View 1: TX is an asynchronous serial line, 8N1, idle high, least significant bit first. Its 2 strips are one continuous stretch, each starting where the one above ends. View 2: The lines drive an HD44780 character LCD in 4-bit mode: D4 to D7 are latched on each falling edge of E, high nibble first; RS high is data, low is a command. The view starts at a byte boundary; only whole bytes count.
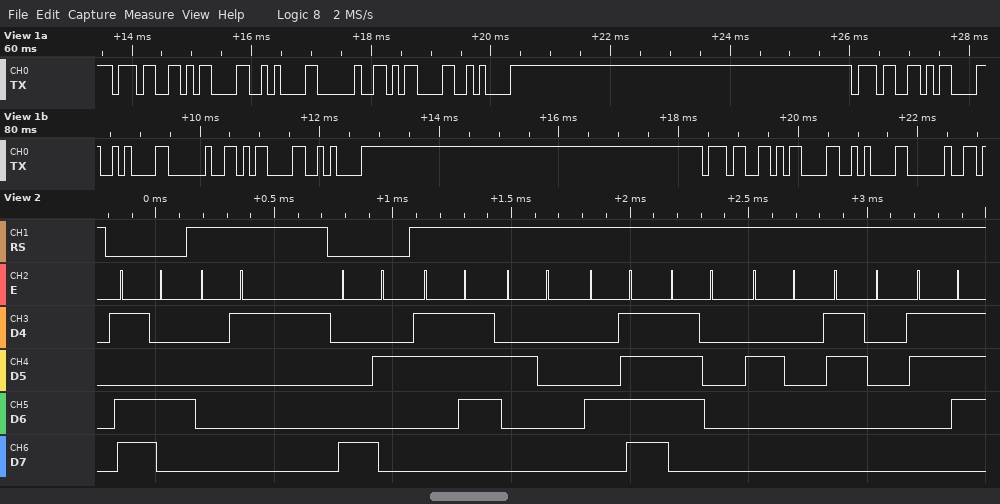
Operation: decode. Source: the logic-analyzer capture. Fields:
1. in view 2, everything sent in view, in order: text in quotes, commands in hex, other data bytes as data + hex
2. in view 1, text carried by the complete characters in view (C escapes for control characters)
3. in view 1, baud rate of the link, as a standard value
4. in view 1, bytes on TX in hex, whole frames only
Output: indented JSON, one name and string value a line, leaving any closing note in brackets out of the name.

{
  "in view 2, everything sent in view, in order: text in quotes, commands in hex, other data bytes as data + hex": "0xD4 data 01 0x82 \"7 Op 07\"",
  "in view 1, text carried by the complete characters in view": "\"7\\r\\n \\r\\n7\\r\\n \\r\\n7\\r\\n \"",
  "in view 1, baud rate of the link, as a standard value": "9600 baud",
  "in view 1, bytes on TX in hex, whole frames only": "0x37 0x0D 0x0A 0x20 0x0D 0x0A 0x37 0x0D 0x0A 0x20 0x0D 0x0A 0x37 0x0D 0x0A 0x20"
}
